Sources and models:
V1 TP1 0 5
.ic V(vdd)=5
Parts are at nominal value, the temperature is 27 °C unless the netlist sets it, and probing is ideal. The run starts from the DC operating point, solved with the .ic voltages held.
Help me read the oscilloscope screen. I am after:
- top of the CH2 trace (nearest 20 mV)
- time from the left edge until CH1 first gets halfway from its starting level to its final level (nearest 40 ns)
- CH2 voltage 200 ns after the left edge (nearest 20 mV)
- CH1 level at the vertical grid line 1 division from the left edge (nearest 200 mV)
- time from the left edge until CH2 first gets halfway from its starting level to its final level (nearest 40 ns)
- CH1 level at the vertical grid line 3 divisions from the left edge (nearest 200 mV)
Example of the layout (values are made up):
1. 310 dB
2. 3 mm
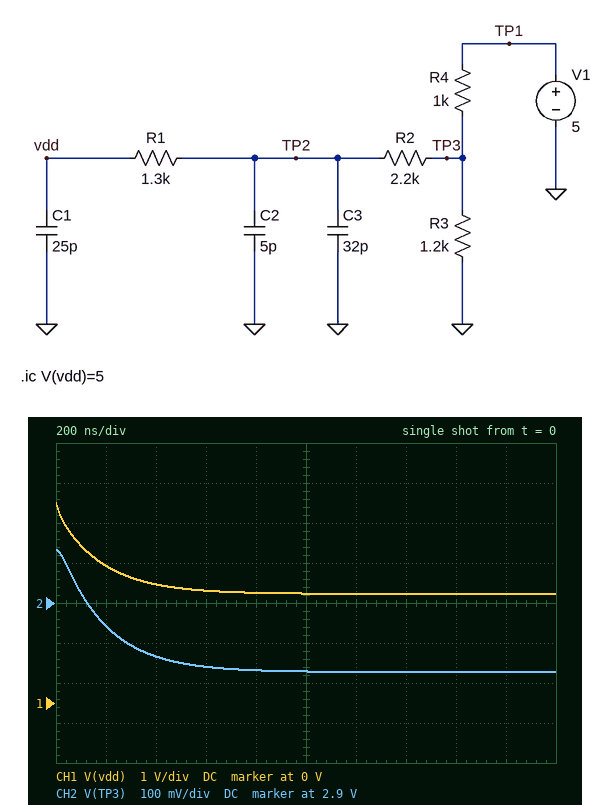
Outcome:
1. 3.04 V
2. 120 ns
3. 2.84 V
4. 3.4 V
5. 160 ns
6. 2.8 V
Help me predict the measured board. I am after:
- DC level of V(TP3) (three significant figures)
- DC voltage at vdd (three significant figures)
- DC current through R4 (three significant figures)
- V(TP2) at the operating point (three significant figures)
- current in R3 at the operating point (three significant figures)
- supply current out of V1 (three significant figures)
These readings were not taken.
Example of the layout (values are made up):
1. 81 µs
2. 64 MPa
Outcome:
1. 2.73 V
2. 2.73 V
3. 2.27 mA
4. 2.73 V
5. 2.27 mA
6. 2.27 mA
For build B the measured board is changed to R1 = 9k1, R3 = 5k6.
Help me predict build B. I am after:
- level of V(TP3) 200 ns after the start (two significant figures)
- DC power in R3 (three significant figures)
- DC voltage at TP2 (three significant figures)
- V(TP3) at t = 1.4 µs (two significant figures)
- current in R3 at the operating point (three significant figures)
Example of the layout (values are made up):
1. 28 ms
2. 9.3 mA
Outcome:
1. 4.3 V
2. 3.21 mW
3. 4.24 V
4. 4.2 V
5. 758 µA
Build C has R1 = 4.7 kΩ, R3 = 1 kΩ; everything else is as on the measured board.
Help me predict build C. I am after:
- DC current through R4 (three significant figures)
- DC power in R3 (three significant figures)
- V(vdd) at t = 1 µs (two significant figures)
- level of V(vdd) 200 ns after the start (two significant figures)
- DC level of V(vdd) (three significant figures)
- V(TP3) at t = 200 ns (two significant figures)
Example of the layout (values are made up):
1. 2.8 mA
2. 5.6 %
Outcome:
1. 2.50 mA
2. 6.25 mW
3. 2.5 V
4. 3.5 V
5. 2.50 V
6. 2.6 V
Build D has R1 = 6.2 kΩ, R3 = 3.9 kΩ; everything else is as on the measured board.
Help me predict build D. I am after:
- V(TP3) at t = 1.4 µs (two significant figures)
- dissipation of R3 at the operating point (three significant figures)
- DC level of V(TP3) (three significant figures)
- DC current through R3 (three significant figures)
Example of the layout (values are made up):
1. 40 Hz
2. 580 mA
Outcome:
1. 4.0 V
2. 4.06 mW
3. 3.98 V
4. 1.02 mA
